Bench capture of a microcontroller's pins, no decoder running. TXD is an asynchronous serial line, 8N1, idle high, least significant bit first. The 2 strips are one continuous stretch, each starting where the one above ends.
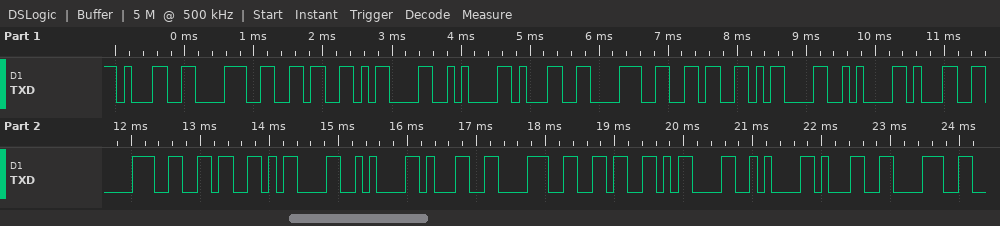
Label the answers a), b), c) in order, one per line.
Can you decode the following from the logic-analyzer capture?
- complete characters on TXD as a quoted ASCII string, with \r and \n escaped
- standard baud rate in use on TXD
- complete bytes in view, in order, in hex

a) "186\r\n186\r\n186\r\n186\r\n18"
b) 9600 baud
c) 31 38 36 0D 0A 31 38 36 0D 0A 31 38 36 0D 0A 31 38 36 0D 0A 31 38
